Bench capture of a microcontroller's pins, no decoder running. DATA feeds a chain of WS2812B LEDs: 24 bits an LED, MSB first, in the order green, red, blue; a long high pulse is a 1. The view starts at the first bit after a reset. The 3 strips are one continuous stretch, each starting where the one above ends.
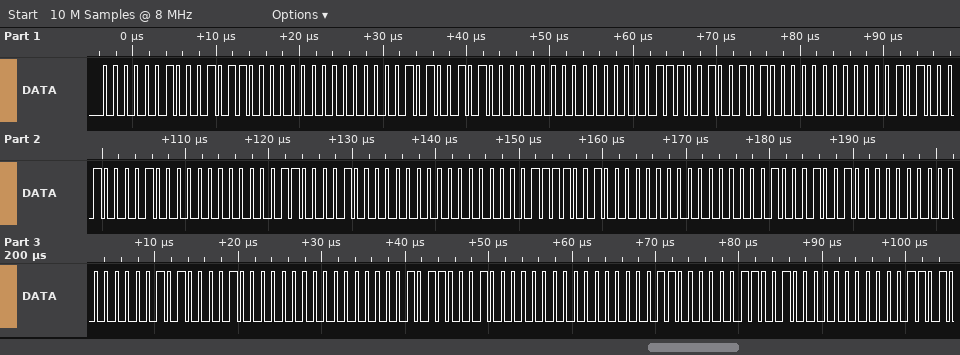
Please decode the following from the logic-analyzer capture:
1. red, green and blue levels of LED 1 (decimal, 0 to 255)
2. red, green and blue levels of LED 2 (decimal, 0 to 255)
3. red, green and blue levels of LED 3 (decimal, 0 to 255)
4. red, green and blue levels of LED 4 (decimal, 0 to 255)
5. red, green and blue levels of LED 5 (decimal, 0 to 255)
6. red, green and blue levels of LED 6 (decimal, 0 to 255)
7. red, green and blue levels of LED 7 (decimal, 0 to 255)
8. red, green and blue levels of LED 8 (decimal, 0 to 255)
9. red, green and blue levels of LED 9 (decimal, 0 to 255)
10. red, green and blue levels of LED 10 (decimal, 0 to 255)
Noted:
44, 2, 0
40, 5, 0
37, 7, 0
33, 10, 0
32, 12, 0
32, 15, 0
32, 17, 0
32, 20, 0
32, 22, 0
25, 24, 0
